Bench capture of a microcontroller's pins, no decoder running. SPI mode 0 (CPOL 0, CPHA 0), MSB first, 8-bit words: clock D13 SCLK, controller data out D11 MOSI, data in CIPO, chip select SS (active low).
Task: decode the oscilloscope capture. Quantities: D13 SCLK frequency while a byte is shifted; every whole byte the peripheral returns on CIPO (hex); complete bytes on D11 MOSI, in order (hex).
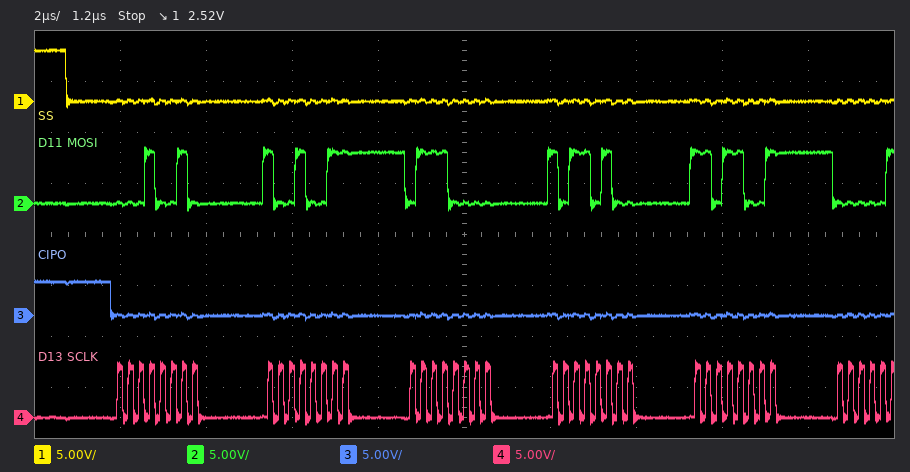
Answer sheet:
4 MHz
00 00 00 00 00
12 93 70 B4 D9
